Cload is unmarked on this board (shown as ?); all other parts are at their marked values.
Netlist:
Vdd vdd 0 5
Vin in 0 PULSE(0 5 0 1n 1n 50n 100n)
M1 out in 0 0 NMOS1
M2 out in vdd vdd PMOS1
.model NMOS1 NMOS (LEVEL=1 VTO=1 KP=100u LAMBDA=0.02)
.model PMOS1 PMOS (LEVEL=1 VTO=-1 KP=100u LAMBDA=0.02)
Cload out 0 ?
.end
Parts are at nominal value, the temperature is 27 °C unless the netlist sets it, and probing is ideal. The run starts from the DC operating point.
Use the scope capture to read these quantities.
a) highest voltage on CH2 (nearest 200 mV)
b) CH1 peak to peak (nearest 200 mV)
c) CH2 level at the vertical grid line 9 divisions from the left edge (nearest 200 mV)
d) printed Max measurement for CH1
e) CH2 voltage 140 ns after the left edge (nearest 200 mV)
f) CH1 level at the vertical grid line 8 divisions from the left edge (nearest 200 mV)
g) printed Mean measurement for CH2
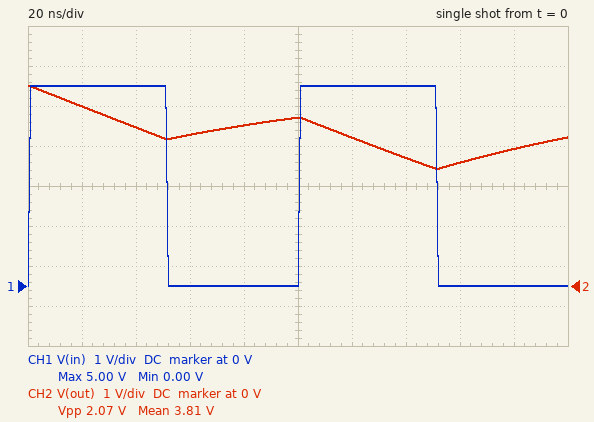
5.0 V
5.0 V
3.4 V
5.00 V
3.2 V
0 V
3.81 V
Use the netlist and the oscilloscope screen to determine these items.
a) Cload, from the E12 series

33 pF
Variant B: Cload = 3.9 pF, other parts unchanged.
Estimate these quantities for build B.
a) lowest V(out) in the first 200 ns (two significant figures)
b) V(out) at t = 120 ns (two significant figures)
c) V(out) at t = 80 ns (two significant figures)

62 mV
1.3 V
4.4 V
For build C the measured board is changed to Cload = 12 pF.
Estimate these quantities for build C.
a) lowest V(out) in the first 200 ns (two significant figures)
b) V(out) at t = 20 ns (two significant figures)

1.2 V
3.6 V
